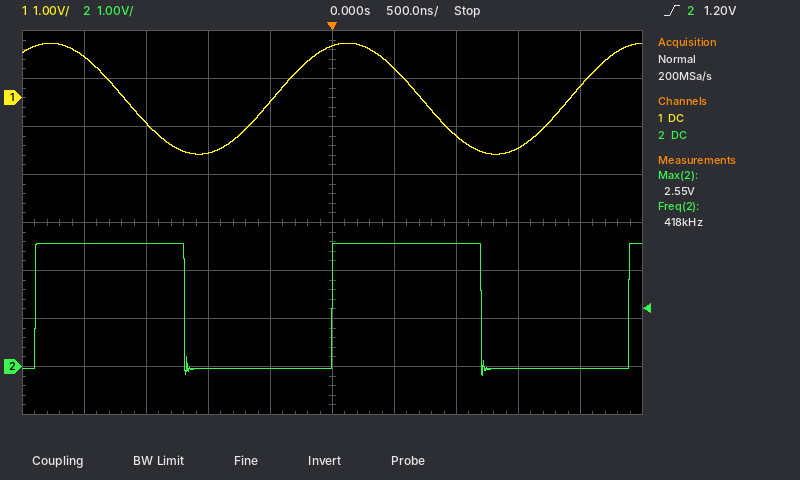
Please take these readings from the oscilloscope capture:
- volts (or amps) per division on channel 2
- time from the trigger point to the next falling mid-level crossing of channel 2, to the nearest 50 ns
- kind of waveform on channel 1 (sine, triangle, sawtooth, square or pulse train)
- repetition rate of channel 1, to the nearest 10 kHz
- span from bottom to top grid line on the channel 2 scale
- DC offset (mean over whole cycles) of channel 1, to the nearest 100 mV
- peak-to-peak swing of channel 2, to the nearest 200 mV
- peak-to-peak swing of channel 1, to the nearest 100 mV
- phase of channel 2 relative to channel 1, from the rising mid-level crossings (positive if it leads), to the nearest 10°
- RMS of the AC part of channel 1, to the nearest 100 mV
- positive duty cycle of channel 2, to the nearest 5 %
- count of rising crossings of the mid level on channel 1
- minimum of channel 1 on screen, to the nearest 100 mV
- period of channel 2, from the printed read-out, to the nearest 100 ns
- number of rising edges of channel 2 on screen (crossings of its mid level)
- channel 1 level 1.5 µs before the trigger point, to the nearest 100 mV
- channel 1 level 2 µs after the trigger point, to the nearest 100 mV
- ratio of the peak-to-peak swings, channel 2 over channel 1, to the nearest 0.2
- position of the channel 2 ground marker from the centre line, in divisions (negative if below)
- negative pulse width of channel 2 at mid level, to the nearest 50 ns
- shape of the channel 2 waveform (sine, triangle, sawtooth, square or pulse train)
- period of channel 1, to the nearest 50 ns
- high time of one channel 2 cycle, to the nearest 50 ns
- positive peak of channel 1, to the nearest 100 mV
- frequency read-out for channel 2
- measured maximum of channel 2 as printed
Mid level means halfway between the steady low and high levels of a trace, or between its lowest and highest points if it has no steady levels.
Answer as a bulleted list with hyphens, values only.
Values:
- 1 V
- 1.20 µs
- sine
- 420 kHz
- 8 V
- 0.0 V
- 2.8 V
- 2.3 V
- -70°
- 800 mV
- 50 %
- 2
- -1.2 V
- 2.4 µs
- 3
- -500 mV
- 200 mV
- 1.2
- -3.0 div
- 1.20 µs
- square
- 2.40 µs
- 1.20 µs
- 1.1 V
- 418 kHz
- 2.55 V
